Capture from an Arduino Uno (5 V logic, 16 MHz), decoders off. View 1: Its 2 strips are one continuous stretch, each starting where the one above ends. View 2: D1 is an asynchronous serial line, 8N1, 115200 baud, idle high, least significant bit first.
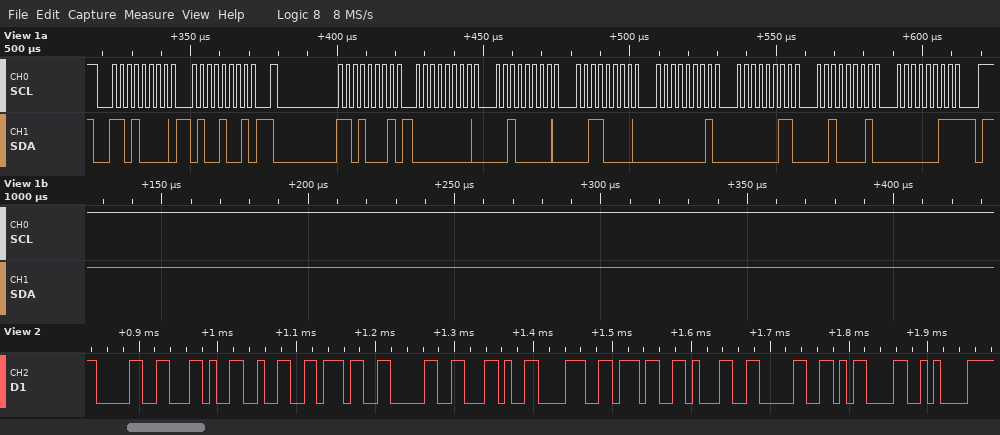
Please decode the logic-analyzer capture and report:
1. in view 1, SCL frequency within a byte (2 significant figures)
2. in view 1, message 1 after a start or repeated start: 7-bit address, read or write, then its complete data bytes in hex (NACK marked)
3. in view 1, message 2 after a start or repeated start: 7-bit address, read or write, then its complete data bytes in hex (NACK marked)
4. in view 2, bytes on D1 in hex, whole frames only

400 kHz
0x68 write: 49
0x68 read: 00 20 30 01 03 21 03 NACK
30 2C 32 37 30 2C 38 37 31 30 0D 0A
